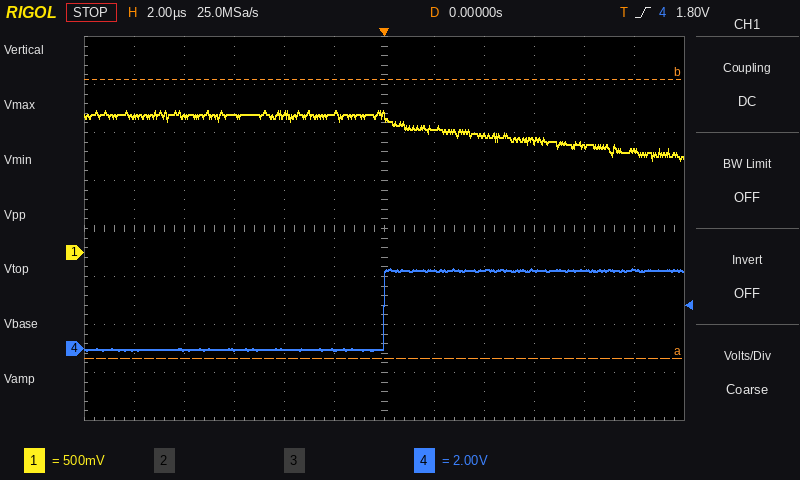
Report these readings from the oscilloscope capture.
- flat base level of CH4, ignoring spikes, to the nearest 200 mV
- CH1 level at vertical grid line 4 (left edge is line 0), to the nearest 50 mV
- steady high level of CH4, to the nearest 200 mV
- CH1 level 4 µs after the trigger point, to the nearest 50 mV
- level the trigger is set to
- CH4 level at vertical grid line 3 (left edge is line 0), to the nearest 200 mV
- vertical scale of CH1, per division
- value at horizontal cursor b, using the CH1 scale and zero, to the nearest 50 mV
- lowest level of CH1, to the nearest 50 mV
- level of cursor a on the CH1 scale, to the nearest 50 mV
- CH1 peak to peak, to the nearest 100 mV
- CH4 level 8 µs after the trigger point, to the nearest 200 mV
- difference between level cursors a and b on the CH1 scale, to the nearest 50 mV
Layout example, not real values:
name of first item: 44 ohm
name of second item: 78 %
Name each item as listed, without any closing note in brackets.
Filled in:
flat base level of CH4, ignoring spikes, to the nearest 200 mV: 0.0 V
CH1 level at vertical grid line 4 (left edge is line 0), to the nearest 50 mV: 1.45 V
steady high level of CH4, to the nearest 200 mV: 3.2 V
CH1 level 4 µs after the trigger point, to the nearest 50 mV: 1.20 V
level the trigger is set to: 1.80 V
CH4 level at vertical grid line 3 (left edge is line 0), to the nearest 200 mV: 0.0 V
vertical scale of CH1, per division: 500 mV
value at horizontal cursor b, using the CH1 scale and zero, to the nearest 50 mV: 1.80 V
lowest level of CH1, to the nearest 50 mV: 950 mV
level of cursor a on the CH1 scale, to the nearest 50 mV: -1.10 V
CH1 peak to peak, to the nearest 100 mV: 500 mV
CH4 level 8 µs after the trigger point, to the nearest 200 mV: 3.2 V
difference between level cursors a and b on the CH1 scale, to the nearest 50 mV: 2.90 V
